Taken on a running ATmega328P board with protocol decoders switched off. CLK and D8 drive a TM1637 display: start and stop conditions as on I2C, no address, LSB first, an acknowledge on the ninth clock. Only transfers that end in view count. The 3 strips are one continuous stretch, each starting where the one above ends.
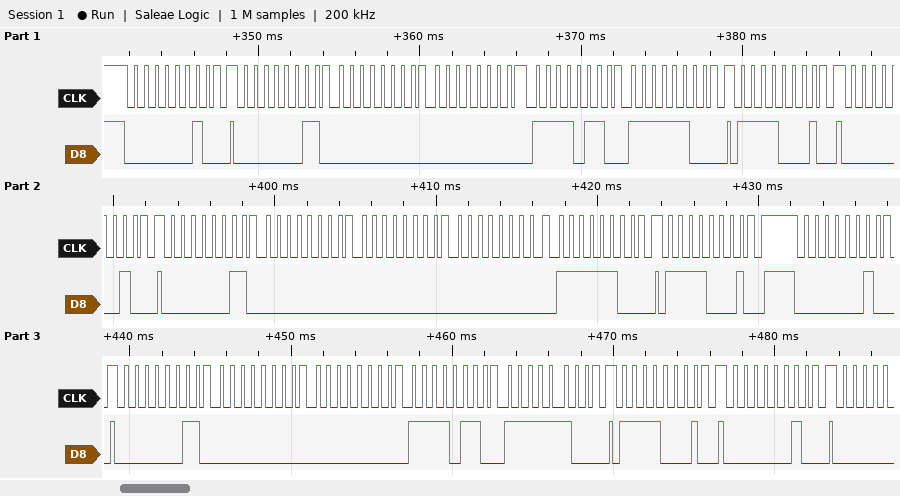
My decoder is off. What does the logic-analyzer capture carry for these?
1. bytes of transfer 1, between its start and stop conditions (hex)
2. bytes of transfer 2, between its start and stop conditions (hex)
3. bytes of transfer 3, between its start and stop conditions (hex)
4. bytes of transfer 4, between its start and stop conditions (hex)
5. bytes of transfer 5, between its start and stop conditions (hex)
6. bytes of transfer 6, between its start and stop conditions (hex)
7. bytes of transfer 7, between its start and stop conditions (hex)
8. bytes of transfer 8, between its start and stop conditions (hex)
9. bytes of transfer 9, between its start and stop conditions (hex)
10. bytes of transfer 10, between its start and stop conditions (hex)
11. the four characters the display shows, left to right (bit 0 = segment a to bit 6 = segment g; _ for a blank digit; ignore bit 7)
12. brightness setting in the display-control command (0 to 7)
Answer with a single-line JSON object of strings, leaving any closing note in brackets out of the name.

{"bytes of transfer 1, between its start and stop conditions": "40", "bytes of transfer 2, between its start and stop conditions": "C0 00 00 6F 3F", "bytes of transfer 3, between its start and stop conditions": "8F", "bytes of transfer 4, between its start and stop conditions": "40", "bytes of transfer 5, between its start and stop conditions": "C0 00 00 00 3F", "bytes of transfer 6, between its start and stop conditions": "8F", "bytes of transfer 7, between its start and stop conditions": "40", "bytes of transfer 8, between its start and stop conditions": "C0 00 00 6F 3F", "bytes of transfer 9, between its start and stop conditions": "8F", "bytes of transfer 10, between its start and stop conditions": "40", "the four characters the display shows, left to right": "__90", "brightness setting in the display-control command": "7"}
